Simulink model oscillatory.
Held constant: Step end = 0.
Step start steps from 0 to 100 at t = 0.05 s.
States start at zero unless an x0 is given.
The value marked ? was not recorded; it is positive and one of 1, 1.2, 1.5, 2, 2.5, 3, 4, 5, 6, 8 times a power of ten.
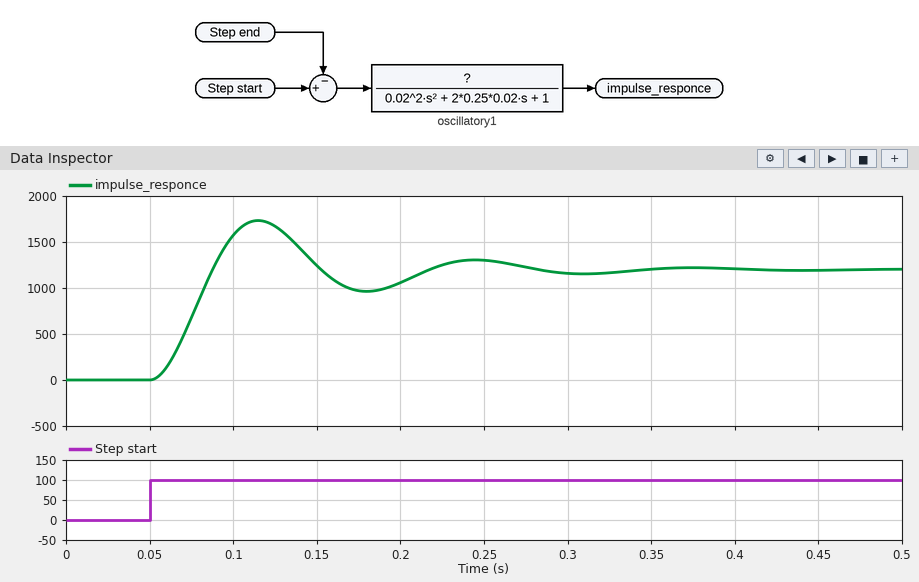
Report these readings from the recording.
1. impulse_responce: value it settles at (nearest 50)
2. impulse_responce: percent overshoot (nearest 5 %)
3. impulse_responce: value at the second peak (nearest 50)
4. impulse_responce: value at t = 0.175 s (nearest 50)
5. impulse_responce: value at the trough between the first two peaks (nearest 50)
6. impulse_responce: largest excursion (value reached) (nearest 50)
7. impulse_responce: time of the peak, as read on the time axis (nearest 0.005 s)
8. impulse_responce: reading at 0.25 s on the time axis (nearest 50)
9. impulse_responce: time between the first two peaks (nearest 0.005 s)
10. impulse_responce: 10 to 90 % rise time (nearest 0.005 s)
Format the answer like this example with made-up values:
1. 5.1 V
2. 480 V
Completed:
1. 1200
2. 45 %
3. 1300
4. 950
5. 950
6. 1750
7. 0.115 s
8. 1300
9. 0.130 s
10. 0.025 s
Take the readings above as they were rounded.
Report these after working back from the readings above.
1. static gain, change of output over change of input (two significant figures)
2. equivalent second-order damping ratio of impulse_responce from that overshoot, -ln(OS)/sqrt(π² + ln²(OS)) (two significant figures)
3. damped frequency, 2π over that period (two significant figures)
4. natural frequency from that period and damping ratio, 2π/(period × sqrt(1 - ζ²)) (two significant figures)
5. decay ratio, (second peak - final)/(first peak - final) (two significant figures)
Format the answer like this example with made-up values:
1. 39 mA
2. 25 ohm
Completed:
1. 12
2. 0.25
3. 48 rad/s
4. 50 rad/s
5. 0.18
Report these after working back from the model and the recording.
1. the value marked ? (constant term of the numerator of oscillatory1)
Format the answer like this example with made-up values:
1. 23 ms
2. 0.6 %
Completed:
1. 12
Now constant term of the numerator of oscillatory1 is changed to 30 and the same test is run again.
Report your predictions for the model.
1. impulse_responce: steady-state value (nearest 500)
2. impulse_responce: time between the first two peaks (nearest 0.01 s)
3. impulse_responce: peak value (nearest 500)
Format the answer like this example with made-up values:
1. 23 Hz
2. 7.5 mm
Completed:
1. 3000
2. 0.13 s
3. 4500
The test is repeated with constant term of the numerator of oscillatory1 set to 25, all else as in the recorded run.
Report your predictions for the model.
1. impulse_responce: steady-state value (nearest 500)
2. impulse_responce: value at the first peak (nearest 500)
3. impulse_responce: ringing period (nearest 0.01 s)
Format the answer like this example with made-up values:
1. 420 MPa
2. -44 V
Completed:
1. 2500
2. 3500
3. 0.13 s
